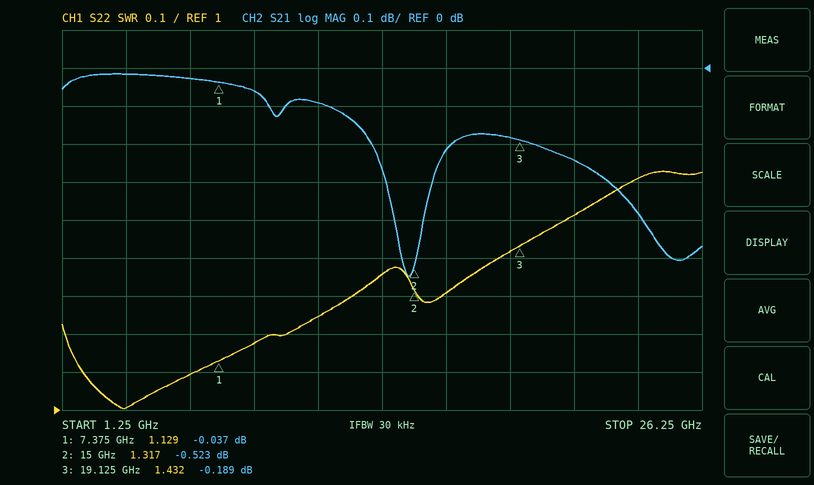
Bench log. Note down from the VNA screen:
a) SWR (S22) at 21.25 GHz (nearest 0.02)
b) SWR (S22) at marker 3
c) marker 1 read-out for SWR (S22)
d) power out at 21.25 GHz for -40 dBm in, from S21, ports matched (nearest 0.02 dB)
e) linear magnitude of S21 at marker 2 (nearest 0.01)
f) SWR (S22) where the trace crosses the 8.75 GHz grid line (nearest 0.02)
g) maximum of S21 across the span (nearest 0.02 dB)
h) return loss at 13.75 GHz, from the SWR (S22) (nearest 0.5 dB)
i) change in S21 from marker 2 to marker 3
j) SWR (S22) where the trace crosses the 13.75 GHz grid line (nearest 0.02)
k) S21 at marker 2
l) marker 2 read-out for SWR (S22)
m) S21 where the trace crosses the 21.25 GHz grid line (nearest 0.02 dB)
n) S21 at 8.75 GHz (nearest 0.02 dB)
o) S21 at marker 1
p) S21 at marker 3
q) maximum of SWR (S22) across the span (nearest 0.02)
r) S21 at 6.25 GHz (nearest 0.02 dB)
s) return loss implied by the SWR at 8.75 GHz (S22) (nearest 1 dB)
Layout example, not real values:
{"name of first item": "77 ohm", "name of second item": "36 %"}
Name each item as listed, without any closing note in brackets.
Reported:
{"SWR (S22) at 21.25 GHz": "1.52", "SWR (S22) at marker 3": "1.432", "marker 1 read-out for SWR": "1.129", "power out at 21.25 GHz for -40 dBm in, from S21, ports matched": "-40.24 dBm", "linear magnitude of S21 at marker 2": "0.94", "SWR (S22) where the trace crosses the 8.75 GHz grid line": "1.18", "maximum of S21 across the span": "-0.02 dB", "return loss at 13.75 GHz, from the SWR (S22)": "16.5 dB", "change in S21 from marker 2 to marker 3": "0.334 dB", "SWR (S22) where the trace crosses the 13.75 GHz grid line": "1.36", "S21 at marker 2": "-0.523 dB", "marker 2 read-out for SWR": "1.317", "S21 where the trace crosses the 21.25 GHz grid line": "-0.24 dB", "S21 at 8.75 GHz": "-0.06 dB", "S21 at marker 1": "-0.037 dB", "S21 at marker 3": "-0.189 dB", "maximum of SWR (S22) across the span": "1.62", "S21 at 6.25 GHz": "-0.02 dB", "return loss implied by the SWR at 8.75 GHz (S22)": "22 dB"}
